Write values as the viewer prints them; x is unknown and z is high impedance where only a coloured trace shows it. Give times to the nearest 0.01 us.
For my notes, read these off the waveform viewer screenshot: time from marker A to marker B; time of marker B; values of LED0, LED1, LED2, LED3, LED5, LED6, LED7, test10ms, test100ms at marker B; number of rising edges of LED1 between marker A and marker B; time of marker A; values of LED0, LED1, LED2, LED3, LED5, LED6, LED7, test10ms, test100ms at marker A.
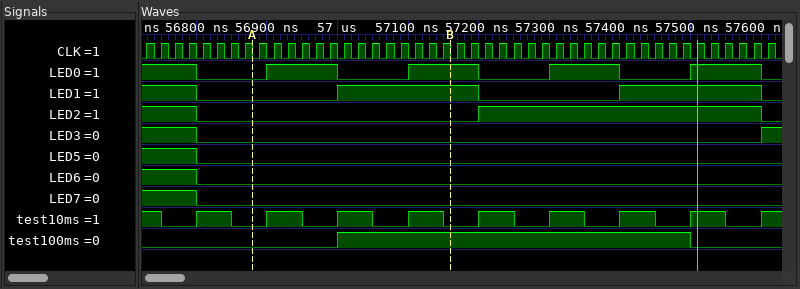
0.28 us
57.16 us
LED0=1, LED1=1, LED2=0, LED3=0, LED5=0, LED6=0, LED7=0, test10ms=0, test100ms=1
1
56.88 us
LED0=0, LED1=0, LED2=0, LED3=0, LED5=0, LED6=0, LED7=0, test10ms=0, test100ms=0
